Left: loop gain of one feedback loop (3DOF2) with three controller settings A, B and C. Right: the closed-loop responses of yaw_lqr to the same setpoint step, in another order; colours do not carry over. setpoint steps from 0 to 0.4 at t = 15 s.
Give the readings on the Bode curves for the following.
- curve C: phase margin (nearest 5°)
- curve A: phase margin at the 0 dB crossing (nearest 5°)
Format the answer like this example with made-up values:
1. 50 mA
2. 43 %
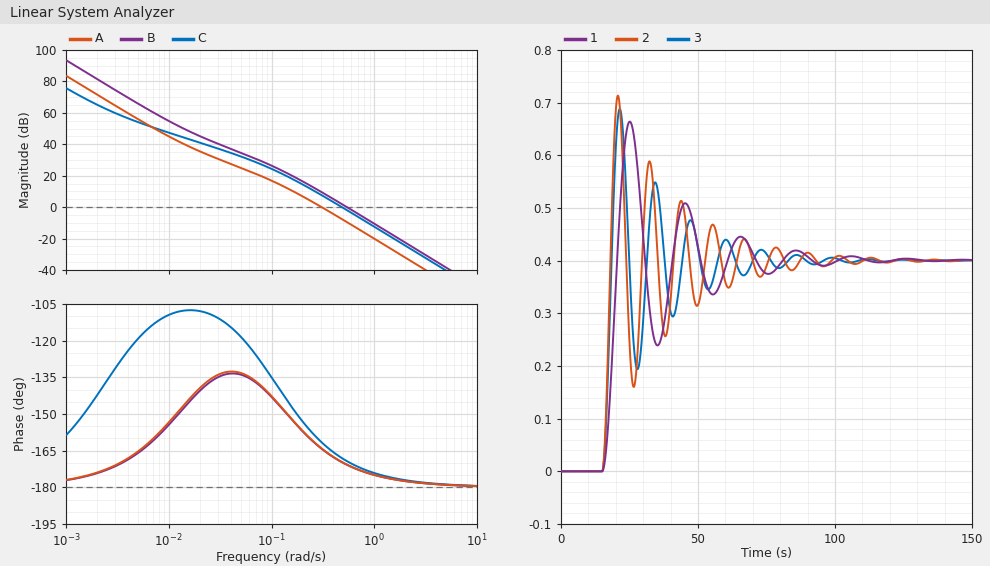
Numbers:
1. 10°
2. 15°
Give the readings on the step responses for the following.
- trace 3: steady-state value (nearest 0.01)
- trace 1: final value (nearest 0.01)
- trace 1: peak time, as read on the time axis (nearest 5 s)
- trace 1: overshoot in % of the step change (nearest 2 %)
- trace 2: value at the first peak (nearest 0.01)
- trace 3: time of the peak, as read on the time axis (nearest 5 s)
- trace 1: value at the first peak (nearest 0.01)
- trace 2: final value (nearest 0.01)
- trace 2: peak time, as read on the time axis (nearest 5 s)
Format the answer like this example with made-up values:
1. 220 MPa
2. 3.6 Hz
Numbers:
1. 0.40
2. 0.40
3. 25 s
4. 66 %
5. 0.71
6. 20 s
7. 0.66
8. 0.40
9. 20 s
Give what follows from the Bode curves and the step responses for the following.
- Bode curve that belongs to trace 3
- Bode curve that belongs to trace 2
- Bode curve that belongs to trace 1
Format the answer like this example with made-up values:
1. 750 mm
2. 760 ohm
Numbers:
1. C
2. B
3. A
